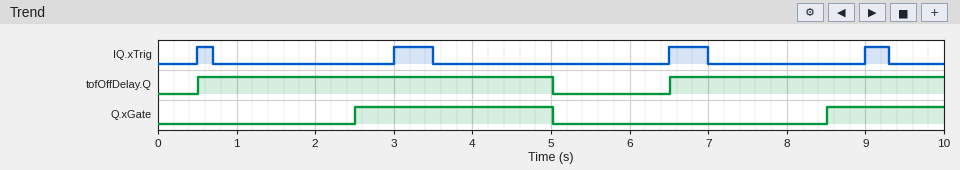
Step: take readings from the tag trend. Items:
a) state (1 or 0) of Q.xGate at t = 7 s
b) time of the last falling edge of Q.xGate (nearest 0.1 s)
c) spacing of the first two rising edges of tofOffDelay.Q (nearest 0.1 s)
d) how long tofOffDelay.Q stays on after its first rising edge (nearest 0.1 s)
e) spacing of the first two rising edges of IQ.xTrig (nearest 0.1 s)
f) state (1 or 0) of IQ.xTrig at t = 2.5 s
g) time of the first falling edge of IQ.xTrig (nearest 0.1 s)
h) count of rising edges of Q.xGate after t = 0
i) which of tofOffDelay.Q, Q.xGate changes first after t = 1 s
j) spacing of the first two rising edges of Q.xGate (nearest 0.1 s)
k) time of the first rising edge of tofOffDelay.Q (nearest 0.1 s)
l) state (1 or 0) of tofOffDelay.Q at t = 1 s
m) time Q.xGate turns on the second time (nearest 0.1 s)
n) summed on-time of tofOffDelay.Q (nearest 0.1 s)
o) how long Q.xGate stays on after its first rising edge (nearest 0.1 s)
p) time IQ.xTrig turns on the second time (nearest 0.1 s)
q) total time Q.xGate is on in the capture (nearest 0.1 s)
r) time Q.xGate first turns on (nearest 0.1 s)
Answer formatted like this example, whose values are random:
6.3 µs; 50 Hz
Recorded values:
0; 5.0 s; 6.0 s; 4.5 s; 2.5 s; 0; 0.7 s; 2; Q.xGate; 6.0 s; 0.5 s; 1; 8.5 s; 8.0 s; 2.5 s; 3.0 s; 4.0 s; 2.5 s
